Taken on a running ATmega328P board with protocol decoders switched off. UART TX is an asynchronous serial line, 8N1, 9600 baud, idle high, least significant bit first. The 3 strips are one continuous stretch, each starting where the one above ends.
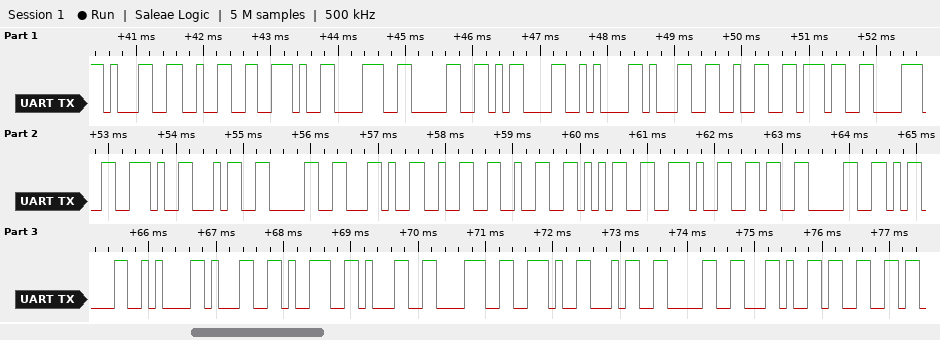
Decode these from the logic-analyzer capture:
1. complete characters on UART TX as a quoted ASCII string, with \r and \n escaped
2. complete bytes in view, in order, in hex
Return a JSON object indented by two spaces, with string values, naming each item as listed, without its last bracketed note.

{
  "complete characters on UART TX as a quoted ASCII string, with \\r and \\n escaped": "\"12.80\\r\\n1278.40,225.60\\r\\n1918.40,3\"",
  "complete bytes in view, in order, in hex": "0x31 0x32 0x2E 0x38 0x30 0x0D 0x0A 0x31 0x32 0x37 0x38 0x2E 0x34 0x30 0x2C 0x32 0x32 0x35 0x2E 0x36 0x30 0x0D 0x0A 0x31 0x39 0x31 0x38 0x2E 0x34 0x30 0x2C 0x33"
}
